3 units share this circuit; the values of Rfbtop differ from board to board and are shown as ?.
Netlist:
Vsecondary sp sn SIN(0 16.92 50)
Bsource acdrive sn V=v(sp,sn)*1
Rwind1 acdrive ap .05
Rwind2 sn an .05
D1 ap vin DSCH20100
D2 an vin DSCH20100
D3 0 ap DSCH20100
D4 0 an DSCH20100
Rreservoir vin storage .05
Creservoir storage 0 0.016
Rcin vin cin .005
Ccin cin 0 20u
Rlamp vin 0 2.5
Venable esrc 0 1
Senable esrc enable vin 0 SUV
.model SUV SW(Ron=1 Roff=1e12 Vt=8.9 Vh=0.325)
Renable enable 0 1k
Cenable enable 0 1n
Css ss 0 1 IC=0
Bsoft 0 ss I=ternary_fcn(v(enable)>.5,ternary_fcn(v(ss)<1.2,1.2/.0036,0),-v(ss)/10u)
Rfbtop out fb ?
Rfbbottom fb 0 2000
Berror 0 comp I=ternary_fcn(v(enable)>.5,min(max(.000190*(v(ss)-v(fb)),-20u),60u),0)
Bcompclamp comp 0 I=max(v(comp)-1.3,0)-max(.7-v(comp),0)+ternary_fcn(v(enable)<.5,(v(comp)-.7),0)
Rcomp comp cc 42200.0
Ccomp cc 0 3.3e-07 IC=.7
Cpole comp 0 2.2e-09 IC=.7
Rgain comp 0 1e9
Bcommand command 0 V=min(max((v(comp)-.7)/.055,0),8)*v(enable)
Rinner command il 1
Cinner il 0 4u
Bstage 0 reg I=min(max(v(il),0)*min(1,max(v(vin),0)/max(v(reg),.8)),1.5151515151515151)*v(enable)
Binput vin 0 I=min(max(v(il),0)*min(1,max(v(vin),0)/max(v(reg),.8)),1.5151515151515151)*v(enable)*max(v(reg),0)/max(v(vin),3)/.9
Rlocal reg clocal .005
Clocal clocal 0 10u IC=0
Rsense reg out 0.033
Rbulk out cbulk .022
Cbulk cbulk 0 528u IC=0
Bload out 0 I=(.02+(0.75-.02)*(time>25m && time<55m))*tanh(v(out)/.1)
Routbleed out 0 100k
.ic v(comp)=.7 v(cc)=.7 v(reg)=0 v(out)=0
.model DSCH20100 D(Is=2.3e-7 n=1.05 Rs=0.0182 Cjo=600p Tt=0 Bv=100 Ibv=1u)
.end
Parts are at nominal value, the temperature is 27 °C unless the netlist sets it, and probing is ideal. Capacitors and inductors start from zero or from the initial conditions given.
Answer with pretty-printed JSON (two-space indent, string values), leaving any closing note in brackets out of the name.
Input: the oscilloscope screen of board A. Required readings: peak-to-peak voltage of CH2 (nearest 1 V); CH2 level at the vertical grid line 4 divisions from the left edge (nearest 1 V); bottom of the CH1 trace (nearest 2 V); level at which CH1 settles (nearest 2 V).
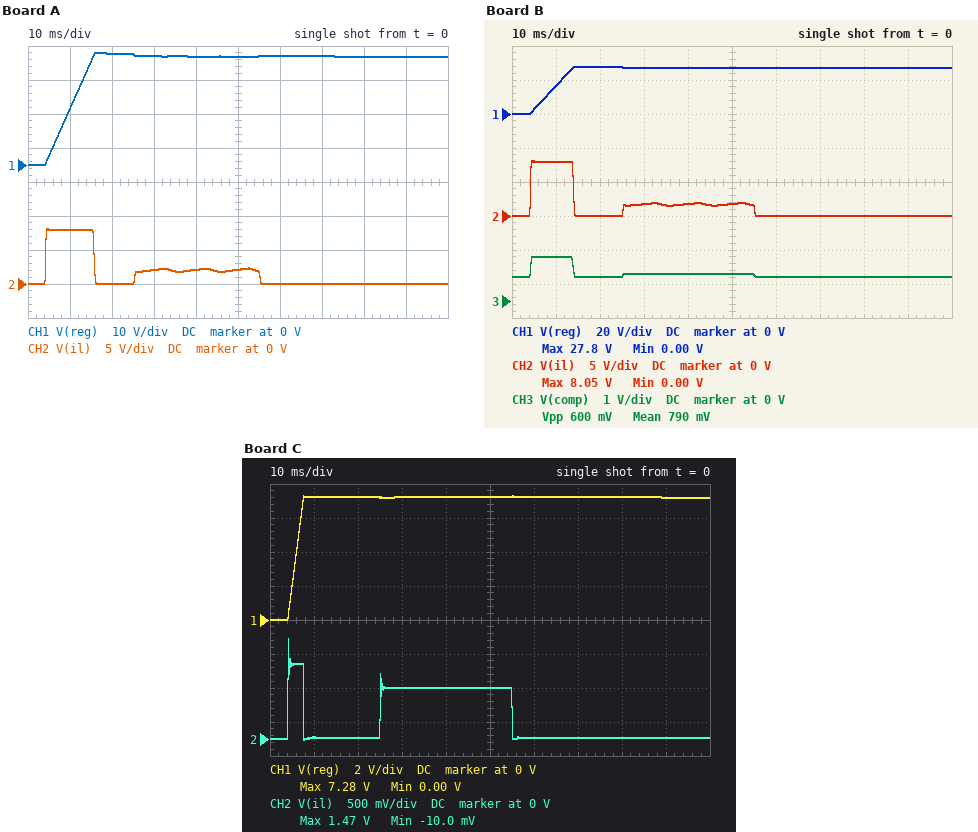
{
  "peak-to-peak voltage of CH2": "8 V",
  "CH2 level at the vertical grid line 4 divisions from the left edge": "2 V",
  "bottom of the CH1 trace": "0 V",
  "level at which CH1 settles": "32 V"
}
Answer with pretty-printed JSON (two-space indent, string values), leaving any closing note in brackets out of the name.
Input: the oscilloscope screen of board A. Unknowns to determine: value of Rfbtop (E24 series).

{
  "value of Rfbtop": "51 kΩ"
}
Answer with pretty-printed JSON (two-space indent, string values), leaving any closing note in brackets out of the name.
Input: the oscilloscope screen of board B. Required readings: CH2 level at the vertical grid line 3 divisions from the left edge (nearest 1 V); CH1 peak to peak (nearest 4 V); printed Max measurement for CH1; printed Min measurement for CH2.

{
  "CH2 level at the vertical grid line 3 divisions from the left edge": "2 V",
  "CH1 peak to peak": "28 V",
  "printed Max measurement for CH1": "27.8 V",
  "printed Min measurement for CH2": "0.00 V"
}
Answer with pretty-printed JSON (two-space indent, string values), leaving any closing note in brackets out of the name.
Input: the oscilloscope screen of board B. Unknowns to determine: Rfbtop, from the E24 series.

{
  "Rfbtop, from the E24 series": "43 kΩ"
}
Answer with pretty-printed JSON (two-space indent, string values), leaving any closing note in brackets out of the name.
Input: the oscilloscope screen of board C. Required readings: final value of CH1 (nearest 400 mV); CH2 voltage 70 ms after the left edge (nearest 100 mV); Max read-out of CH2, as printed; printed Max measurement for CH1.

{
  "final value of CH1": "7.2 V",
  "CH2 voltage 70 ms after the left edge": "0 V",
  "Max read-out of CH2, as printed": "1.47 V",
  "printed Max measurement for CH1": "7.28 V"
}
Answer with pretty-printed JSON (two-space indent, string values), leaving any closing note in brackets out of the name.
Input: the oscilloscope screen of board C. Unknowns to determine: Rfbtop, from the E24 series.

{
  "Rfbtop, from the E24 series": "10 kΩ"
}
